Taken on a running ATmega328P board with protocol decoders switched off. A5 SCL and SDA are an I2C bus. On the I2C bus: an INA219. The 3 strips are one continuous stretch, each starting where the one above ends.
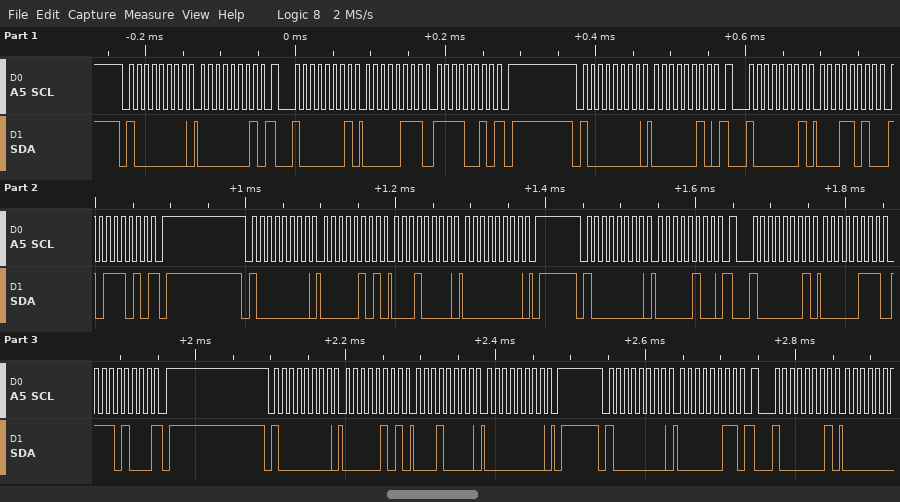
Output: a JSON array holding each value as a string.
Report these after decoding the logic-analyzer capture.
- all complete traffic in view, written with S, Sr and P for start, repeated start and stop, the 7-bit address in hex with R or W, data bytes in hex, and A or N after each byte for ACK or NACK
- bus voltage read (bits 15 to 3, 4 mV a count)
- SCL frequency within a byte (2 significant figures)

["S 40W A 01 A Sr 40R A 07 A F2 N P S 40W A 02 A Sr 40R A 1A A BA N P S 40W A 05 A 10 A 00 A P S 40W A 04 A Sr 40R A 07 A E8 N P S 40W A 05 A 10 A 00 A P S 40W A 03 A Sr 40R A", "3.420 V", "100 kHz"]
